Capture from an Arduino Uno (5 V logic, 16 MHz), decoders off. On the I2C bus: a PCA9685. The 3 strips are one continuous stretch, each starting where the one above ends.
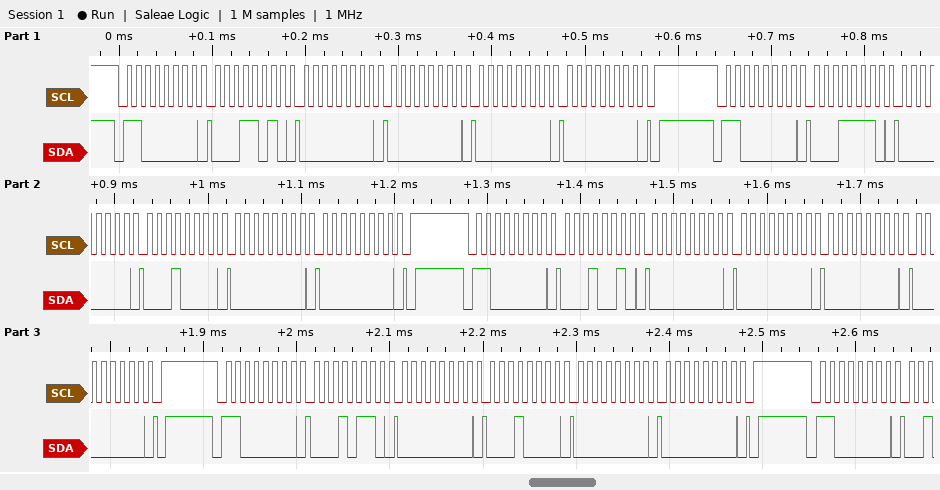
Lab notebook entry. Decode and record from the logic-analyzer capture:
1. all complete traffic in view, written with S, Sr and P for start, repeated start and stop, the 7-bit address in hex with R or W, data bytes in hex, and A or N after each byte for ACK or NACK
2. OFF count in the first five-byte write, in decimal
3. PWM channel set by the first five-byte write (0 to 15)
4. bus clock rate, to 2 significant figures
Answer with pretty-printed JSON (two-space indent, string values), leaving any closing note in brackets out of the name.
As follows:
{
  "all complete traffic in view, written with S, Sr and P for start, repeated start and stop, the 7-bit address in hex with R or W, data bytes in hex, and A or N after each byte for ACK or NACK": "S 60W A 1A A 00 A 00 A 00 A 00 A P S 60W A 1E A 00 A 10 A 00 A 00 A P S 60W A 12 A 00 A 00 A 00 A 00 A P S 60W A 16 A 00 A 10 A 00 A 00 A P S 60W A",
  "OFF count in the first five-byte write, in decimal": "0",
  "PWM channel set by the first five-byte write": "5",
  "bus clock rate, to 2 significant figures": "100 kHz"
}
